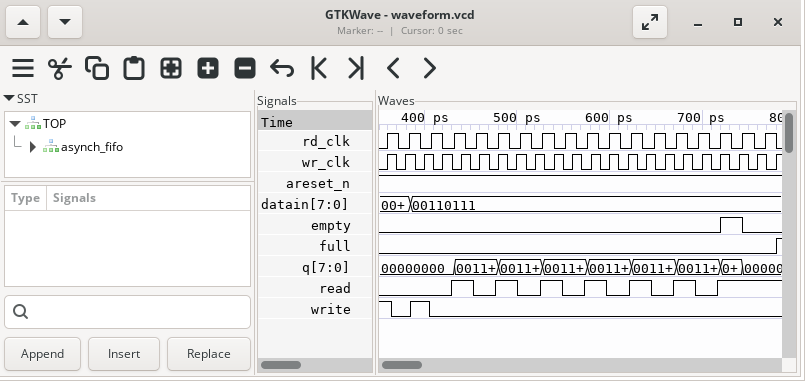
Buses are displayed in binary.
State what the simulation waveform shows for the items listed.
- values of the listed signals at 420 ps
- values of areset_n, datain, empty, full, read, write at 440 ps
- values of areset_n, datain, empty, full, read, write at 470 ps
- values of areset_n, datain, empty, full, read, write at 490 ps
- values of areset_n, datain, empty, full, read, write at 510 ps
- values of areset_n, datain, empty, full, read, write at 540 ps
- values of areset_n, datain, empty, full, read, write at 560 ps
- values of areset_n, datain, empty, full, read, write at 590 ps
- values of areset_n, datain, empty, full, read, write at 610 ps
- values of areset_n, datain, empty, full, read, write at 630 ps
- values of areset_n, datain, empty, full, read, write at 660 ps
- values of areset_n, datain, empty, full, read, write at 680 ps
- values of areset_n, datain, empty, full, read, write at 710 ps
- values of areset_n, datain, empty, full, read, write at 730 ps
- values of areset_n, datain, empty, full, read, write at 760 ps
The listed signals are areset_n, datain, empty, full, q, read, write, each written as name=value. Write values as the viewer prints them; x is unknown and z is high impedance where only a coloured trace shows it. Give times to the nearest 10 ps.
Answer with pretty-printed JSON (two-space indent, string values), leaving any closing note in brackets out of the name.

{
  "values of the listed signals at 420 ps": "areset_n=1, datain=00110111, empty=0, full=0, q=00000000, read=0, write=0",
  "values of areset_n, datain, empty, full, read, write at 440 ps": "areset_n=1, datain=00110111, empty=0, full=0, read=1, write=0",
  "values of areset_n, datain, empty, full, read, write at 470 ps": "areset_n=1, datain=00110111, empty=0, full=0, read=0, write=0",
  "values of areset_n, datain, empty, full, read, write at 490 ps": "areset_n=1, datain=00110111, empty=0, full=0, read=1, write=0",
  "values of areset_n, datain, empty, full, read, write at 510 ps": "areset_n=1, datain=00110111, empty=0, full=0, read=0, write=0",
  "values of areset_n, datain, empty, full, read, write at 540 ps": "areset_n=1, datain=00110111, empty=0, full=0, read=1, write=0",
  "values of areset_n, datain, empty, full, read, write at 560 ps": "areset_n=1, datain=00110111, empty=0, full=0, read=0, write=0",
  "values of areset_n, datain, empty, full, read, write at 590 ps": "areset_n=1, datain=00110111, empty=0, full=0, read=1, write=0",
  "values of areset_n, datain, empty, full, read, write at 610 ps": "areset_n=1, datain=00110111, empty=0, full=0, read=0, write=0",
  "values of areset_n, datain, empty, full, read, write at 630 ps": "areset_n=1, datain=00110111, empty=0, full=0, read=1, write=0",
  "values of areset_n, datain, empty, full, read, write at 660 ps": "areset_n=1, datain=00110111, empty=0, full=0, read=0, write=0",
  "values of areset_n, datain, empty, full, read, write at 680 ps": "areset_n=1, datain=00110111, empty=0, full=0, read=1, write=0",
  "values of areset_n, datain, empty, full, read, write at 710 ps": "areset_n=1, datain=00110111, empty=0, full=0, read=0, write=0",
  "values of areset_n, datain, empty, full, read, write at 730 ps": "areset_n=1, datain=00110111, empty=1, full=0, read=1, write=0",
  "values of areset_n, datain, empty, full, read, write at 760 ps": "areset_n=1, datain=00110111, empty=0, full=0, read=1, write=0"
}
